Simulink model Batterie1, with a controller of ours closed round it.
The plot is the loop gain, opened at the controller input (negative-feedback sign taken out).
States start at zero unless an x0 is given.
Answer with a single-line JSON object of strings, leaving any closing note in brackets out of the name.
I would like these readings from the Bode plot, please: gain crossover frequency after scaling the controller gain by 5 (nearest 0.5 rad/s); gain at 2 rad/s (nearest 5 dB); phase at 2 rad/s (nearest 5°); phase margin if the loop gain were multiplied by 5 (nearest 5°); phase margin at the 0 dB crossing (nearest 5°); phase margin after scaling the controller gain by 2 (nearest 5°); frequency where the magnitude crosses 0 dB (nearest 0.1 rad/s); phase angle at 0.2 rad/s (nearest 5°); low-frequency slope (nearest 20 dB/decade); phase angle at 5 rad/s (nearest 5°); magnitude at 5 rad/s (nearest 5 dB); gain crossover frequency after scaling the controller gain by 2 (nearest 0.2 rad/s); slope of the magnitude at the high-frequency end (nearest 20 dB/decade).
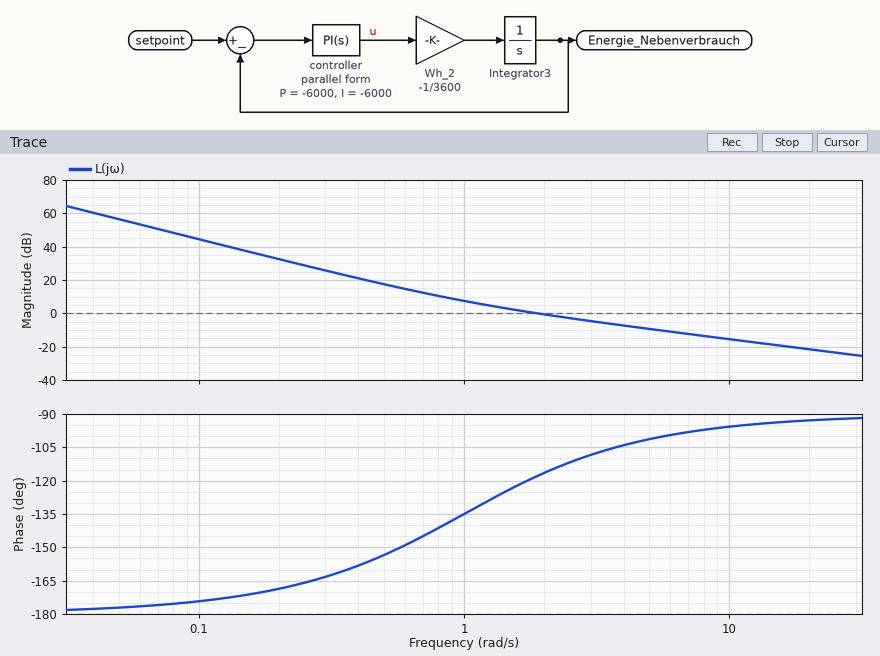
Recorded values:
{"gain crossover frequency after scaling the controller gain by 5": "8.5 rad/s", "gain at 2 rad/s": "0 dB", "phase at 2 rad/s": "-115°", "phase margin if the loop gain were multiplied by 5": "85°", "phase margin at the 0 dB crossing": "60°", "phase margin after scaling the controller gain by 2": "75°", "frequency where the magnitude crosses 0 dB": "1.9 rad/s", "phase angle at 0.2 rad/s": "-170°", "low-frequency slope": "-40 dB/decade", "phase angle at 5 rad/s": "-100°", "magnitude at 5 rad/s": "-10 dB", "gain crossover frequency after scaling the controller gain by 2": "3.4 rad/s", "slope of the magnitude at the high-frequency end": "-20 dB/decade"}
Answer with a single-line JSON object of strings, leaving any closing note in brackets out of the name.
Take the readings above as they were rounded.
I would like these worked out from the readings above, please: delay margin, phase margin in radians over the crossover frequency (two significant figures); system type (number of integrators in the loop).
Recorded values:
{"delay margin, phase margin in radians over the crossover frequency": "0.55 s", "system type": "2"}
